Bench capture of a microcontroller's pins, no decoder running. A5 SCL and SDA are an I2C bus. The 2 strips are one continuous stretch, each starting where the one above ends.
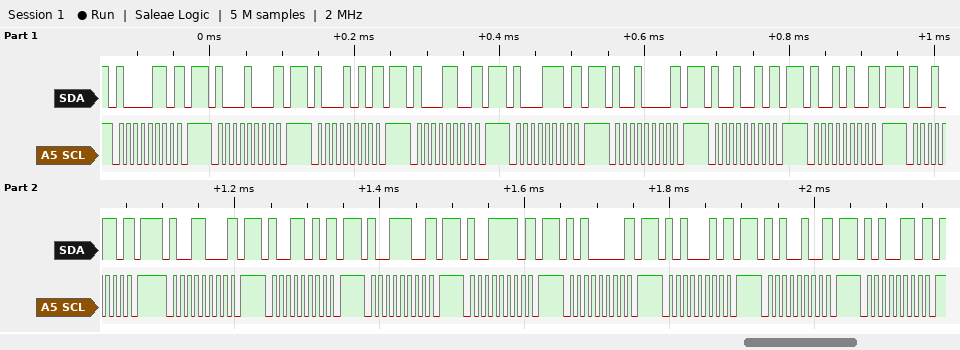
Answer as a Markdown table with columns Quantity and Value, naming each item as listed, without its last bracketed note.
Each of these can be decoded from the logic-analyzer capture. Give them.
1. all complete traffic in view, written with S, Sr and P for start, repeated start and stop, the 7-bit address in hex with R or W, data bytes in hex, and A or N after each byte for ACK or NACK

| Quantity | Value |
|---|---|
| all complete traffic in view, written with S, Sr and P for start, repeated start and stop, the 7-bit address in hex with R or W, data bytes in hex, and A or N after each byte for ACK or NACK | S 43W N P S 44W N P S 45W N P S 46W N P S 47W N P S 48W N P S 49W N P S 4AW N P S 4BW N P S 4CW N P S 4DW N P S 4EW N P S 4FW N P S 50W N P S 51W N P S 52W N P S 53W N P |
